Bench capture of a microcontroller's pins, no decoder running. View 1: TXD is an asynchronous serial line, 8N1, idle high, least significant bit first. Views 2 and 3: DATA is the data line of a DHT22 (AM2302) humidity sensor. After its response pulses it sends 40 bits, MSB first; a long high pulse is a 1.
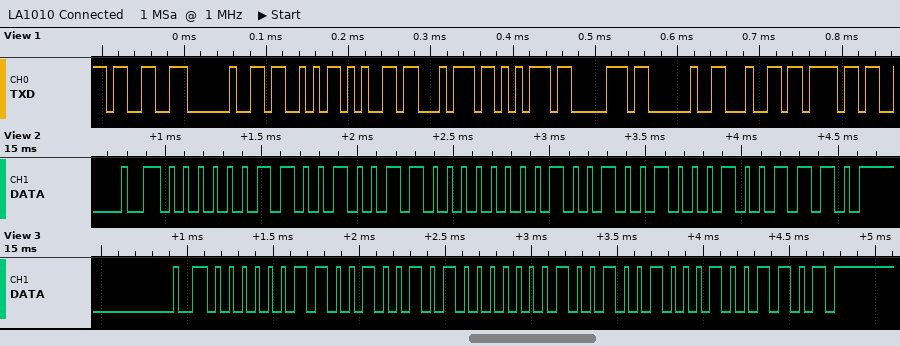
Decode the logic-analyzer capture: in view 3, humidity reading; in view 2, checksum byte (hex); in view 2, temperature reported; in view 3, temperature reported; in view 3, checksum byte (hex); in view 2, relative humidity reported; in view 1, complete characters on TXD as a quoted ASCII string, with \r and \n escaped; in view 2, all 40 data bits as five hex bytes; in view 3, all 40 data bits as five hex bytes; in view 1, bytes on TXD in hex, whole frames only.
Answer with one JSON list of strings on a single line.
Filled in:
["80.5 %", "0x4E", "29.2 °C", "29.2 °C", "0x4D", "80.6 %", "\"3 Setup do\"", "03 26 01 24 4E", "03 25 01 24 4D", "0x33 0x20 0x53 0x65 0x74 0x75 0x70 0x20 0x64 0x6F"]
